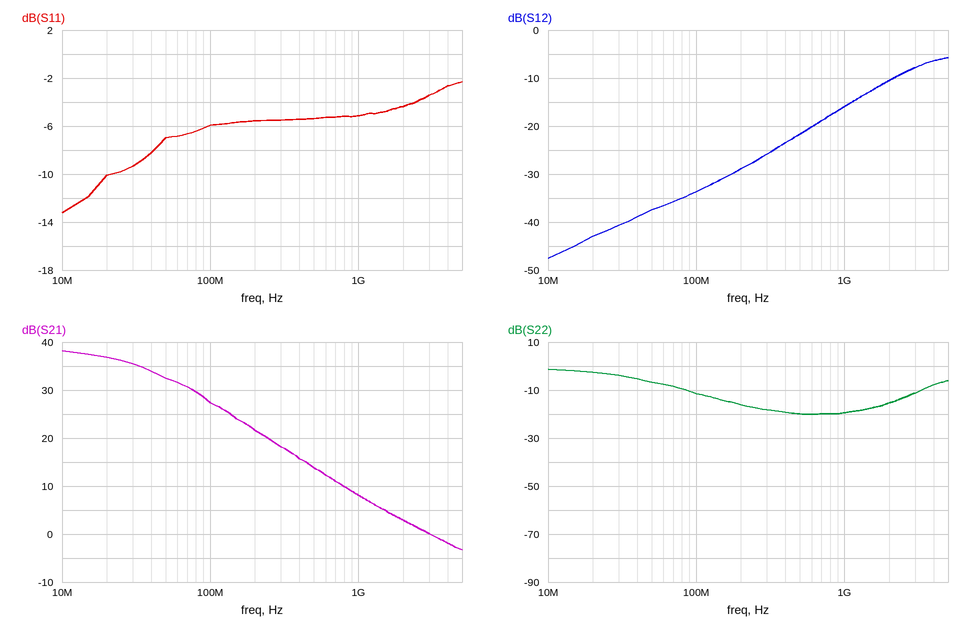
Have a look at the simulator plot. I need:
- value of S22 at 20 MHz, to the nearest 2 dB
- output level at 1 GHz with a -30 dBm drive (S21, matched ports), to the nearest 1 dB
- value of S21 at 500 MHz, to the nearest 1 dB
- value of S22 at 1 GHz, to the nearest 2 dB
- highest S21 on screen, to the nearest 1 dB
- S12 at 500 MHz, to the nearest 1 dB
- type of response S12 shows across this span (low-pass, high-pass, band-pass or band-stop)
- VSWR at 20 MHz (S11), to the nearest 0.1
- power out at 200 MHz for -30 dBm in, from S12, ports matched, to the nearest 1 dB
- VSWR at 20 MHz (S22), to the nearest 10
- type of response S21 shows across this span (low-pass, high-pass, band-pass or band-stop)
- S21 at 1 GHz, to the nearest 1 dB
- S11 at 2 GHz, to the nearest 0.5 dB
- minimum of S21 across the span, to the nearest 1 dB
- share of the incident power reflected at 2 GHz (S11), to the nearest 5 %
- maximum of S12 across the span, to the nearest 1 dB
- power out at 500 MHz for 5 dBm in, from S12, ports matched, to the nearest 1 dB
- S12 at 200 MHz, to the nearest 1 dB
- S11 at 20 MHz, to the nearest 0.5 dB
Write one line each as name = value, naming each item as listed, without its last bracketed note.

value of S22 at 20 MHz, to the nearest 2 dB = -2 dB
output level at 1 GHz with a -30 dBm drive (S21, matched ports), to the nearest 1 dB = -22 dBm
value of S21 at 500 MHz, to the nearest 1 dB = 14 dB
value of S22 at 1 GHz, to the nearest 2 dB = -20 dB
highest S21 on screen, to the nearest 1 dB = 38 dB
S12 at 500 MHz, to the nearest 1 dB = -22 dB
type of response S12 shows across this span = high-pass
VSWR at 20 MHz (S11), to the nearest 0.1 = 1.9
power out at 200 MHz for -30 dBm in, from S12, ports matched, to the nearest 1 dB = -59 dBm
VSWR at 20 MHz (S22), to the nearest 10 = 10
type of response S21 shows across this span = low-pass
S21 at 1 GHz, to the nearest 1 dB = 8 dB
S11 at 2 GHz, to the nearest 0.5 dB = -4.5 dB
minimum of S21 across the span, to the nearest 1 dB = -3 dB
share of the incident power reflected at 2 GHz (S11), to the nearest 5 % = 35 %
maximum of S12 across the span, to the nearest 1 dB = -6 dB
power out at 500 MHz for 5 dBm in, from S12, ports matched, to the nearest 1 dB = -17 dBm
S12 at 200 MHz, to the nearest 1 dB = -29 dB
S11 at 20 MHz, to the nearest 0.5 dB = -10.0 dB
